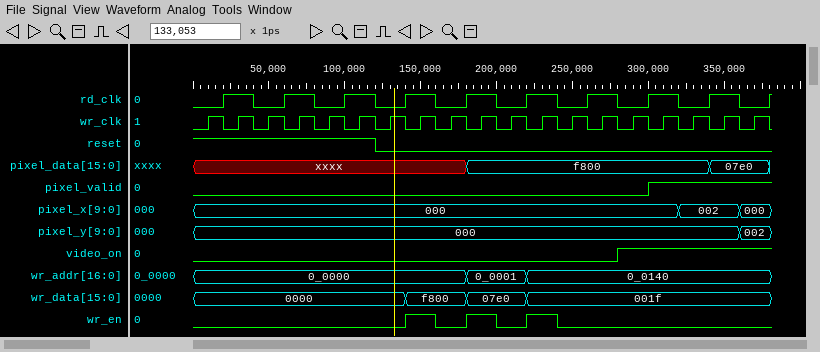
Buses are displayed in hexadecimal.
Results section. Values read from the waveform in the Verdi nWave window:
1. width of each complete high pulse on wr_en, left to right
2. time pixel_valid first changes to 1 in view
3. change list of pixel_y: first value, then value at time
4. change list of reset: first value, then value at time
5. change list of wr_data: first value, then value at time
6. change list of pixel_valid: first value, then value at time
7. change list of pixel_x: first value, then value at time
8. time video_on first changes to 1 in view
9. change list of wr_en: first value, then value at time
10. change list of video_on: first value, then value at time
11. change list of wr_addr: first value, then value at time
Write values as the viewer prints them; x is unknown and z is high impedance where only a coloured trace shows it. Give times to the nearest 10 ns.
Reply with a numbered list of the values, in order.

1. 20 ns, 20 ns, 20 ns
2. 300 ns
3. 000, 002 at 360 ns
4. 1, 0 at 120 ns
5. 0000, f800 at 140 ns, 07e0 at 180 ns, 001f at 220 ns
6. 0, 1 at 300 ns
7. 000, 002 at 320 ns, 000 at 360 ns
8. 280 ns
9. 0, 1 at 140 ns, 0 at 160 ns, 1 at 180 ns, 0 at 200 ns, 1 at 220 ns, 0 at 240 ns
10. 0, 1 at 280 ns
11. 0_0000, 0_0001 at 180 ns, 0_0140 at 220 ns
